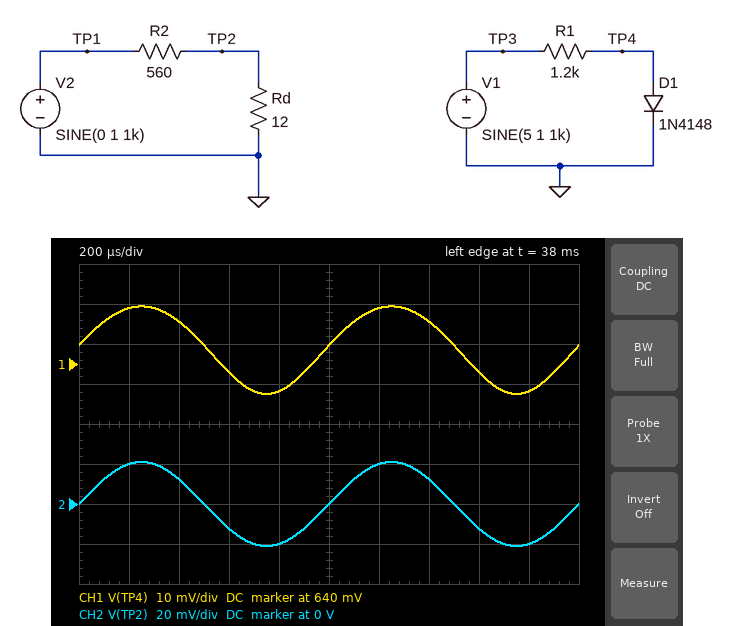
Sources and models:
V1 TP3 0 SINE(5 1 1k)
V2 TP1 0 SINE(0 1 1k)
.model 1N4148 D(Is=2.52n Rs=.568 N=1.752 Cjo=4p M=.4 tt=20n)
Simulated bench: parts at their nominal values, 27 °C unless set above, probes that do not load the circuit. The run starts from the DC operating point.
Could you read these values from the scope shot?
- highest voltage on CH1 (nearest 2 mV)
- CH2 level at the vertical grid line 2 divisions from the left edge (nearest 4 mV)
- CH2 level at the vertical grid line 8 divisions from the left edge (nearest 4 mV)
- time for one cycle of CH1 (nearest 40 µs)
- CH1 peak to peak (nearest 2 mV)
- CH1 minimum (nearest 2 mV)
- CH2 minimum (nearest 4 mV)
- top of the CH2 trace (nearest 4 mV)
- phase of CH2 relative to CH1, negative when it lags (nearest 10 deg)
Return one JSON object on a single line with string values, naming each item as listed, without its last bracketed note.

{"highest voltage on CH1": "654 mV", "CH2 level at the vertical grid line 2 divisions from the left edge": "12 mV", "CH2 level at the vertical grid line 8 divisions from the left edge": "-12 mV", "time for one cycle of CH1": "1.00 ms", "CH1 peak to peak": "22 mV", "CH1 minimum": "632 mV", "CH2 minimum": "-20 mV", "top of the CH2 trace": "20 mV", "phase of CH2 relative to CH1, negative when it lags": "0 deg"}
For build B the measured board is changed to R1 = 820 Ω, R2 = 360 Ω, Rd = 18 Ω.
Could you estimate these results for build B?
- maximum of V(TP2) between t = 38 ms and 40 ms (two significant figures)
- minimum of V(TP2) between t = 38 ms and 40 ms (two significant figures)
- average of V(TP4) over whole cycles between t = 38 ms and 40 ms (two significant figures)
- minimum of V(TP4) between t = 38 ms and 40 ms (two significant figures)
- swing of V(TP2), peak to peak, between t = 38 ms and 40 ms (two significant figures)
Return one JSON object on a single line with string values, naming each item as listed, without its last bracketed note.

{"maximum of V(TP2) between t = 38 ms and 40 ms": "48 mV", "minimum of V(TP2) between t = 38 ms and 40 ms": "-48 mV", "average of V(TP4) over whole cycles between t = 38 ms and 40 ms": "660 mV", "minimum of V(TP4) between t = 38 ms and 40 ms": "650 mV", "swing of V(TP2), peak to peak, between t = 38 ms and 40 ms": "95 mV"}
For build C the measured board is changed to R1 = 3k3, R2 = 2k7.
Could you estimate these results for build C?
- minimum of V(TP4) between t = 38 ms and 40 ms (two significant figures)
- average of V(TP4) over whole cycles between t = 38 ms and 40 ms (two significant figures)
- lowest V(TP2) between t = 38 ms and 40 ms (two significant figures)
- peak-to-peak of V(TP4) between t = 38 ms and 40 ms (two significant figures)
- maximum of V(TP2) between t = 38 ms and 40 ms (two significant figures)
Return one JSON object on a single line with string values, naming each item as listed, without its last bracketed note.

{"minimum of V(TP4) between t = 38 ms and 40 ms": "590 mV", "average of V(TP4) over whole cycles between t = 38 ms and 40 ms": "600 mV", "lowest V(TP2) between t = 38 ms and 40 ms": "-4.4 mV", "peak-to-peak of V(TP4) between t = 38 ms and 40 ms": "21 mV", "maximum of V(TP2) between t = 38 ms and 40 ms": "4.4 mV"}
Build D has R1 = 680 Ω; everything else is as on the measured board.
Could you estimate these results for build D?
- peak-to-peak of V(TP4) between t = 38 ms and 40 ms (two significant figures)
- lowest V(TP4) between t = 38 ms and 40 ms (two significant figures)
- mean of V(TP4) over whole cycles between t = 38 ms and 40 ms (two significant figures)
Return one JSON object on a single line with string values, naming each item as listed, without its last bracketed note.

{"peak-to-peak of V(TP4) between t = 38 ms and 40 ms": "23 mV", "lowest V(TP4) between t = 38 ms and 40 ms": "660 mV", "mean of V(TP4) over whole cycles between t = 38 ms and 40 ms": "670 mV"}
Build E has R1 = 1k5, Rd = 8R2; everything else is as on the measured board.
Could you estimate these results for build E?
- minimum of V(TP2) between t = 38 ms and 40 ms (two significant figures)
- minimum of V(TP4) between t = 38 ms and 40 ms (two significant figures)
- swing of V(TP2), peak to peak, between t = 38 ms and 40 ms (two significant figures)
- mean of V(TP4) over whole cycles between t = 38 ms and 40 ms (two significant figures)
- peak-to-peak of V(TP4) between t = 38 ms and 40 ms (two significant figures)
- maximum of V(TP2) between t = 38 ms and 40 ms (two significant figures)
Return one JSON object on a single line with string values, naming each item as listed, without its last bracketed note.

{"minimum of V(TP2) between t = 38 ms and 40 ms": "-14 mV", "minimum of V(TP4) between t = 38 ms and 40 ms": "620 mV", "swing of V(TP2), peak to peak, between t = 38 ms and 40 ms": "29 mV", "mean of V(TP4) over whole cycles between t = 38 ms and 40 ms": "630 mV", "peak-to-peak of V(TP4) between t = 38 ms and 40 ms": "22 mV", "maximum of V(TP2) between t = 38 ms and 40 ms": "14 mV"}
